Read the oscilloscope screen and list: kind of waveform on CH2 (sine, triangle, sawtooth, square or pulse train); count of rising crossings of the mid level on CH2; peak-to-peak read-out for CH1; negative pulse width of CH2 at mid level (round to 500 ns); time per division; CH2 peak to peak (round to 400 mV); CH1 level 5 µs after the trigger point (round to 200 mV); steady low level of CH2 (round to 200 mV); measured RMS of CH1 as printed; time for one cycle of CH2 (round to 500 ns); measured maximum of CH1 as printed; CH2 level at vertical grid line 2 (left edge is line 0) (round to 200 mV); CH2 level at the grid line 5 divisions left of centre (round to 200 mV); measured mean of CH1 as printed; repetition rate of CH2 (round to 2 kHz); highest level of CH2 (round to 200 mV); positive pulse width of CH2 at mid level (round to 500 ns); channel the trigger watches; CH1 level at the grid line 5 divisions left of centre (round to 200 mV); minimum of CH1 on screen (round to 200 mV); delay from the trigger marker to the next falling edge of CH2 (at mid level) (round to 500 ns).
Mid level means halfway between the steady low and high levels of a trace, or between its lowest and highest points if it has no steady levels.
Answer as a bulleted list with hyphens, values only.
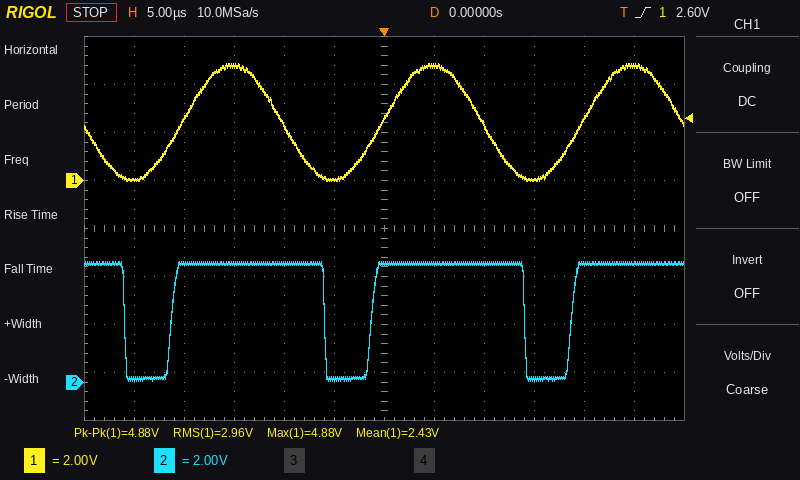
- pulse train
- 3
- 4.88 V
- 4.5 µs
- 5 µs
- 4.8 V
- 4.8 V
- 200 mV
- 2.96 V
- 20.0 µs
- 4.88 V
- 5.0 V
- 200 mV
- 2.43 V
- 50 kHz
- 5.0 V
- 15.5 µs
- CH1
- 0.0 V
- 0.0 V
- 14.0 µs
